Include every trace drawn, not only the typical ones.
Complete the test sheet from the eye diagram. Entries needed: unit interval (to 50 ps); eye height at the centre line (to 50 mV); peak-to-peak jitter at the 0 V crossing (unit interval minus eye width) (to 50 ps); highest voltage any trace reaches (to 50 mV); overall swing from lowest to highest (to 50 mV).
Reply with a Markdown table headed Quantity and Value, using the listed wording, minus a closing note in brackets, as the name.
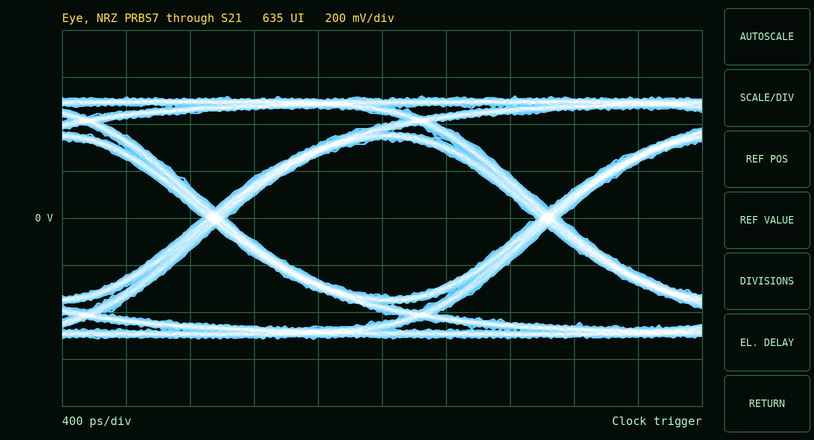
| Quantity | Value |
|---|---|
| unit interval | 2.10 ns |
| eye height at the centre line | 650 mV |
| peak-to-peak jitter at the 0 V crossing (unit interval minus eye width) | 150 ps |
| highest voltage any trace reaches | 500 mV |
| overall swing from lowest to highest | 1.05 V |
